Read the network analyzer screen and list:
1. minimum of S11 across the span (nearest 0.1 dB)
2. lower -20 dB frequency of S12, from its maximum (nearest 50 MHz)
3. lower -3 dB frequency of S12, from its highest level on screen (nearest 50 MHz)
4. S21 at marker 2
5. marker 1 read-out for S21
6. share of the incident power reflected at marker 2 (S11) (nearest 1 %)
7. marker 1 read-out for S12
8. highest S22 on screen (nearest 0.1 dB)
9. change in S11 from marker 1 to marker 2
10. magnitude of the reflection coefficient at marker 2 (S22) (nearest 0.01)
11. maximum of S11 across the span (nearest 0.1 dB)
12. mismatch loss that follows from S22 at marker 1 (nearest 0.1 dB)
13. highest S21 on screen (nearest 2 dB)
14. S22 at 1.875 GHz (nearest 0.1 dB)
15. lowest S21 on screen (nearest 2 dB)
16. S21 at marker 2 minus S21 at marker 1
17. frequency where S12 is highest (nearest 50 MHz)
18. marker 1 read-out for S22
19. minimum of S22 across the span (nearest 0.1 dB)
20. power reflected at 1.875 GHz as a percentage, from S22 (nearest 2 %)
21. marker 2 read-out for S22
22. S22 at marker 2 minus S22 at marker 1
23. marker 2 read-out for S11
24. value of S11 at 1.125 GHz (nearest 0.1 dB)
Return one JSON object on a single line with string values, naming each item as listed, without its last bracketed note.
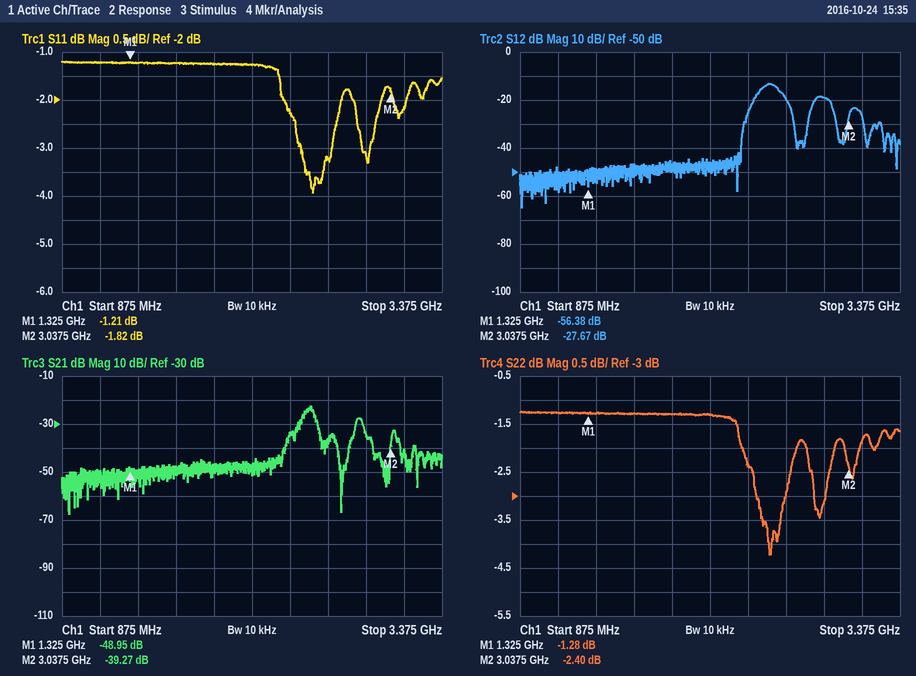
{"minimum of S11 across the span": "-3.9 dB", "lower -20 dB frequency of S12, from its maximum": "2.35 GHz", "lower -3 dB frequency of S12, from its highest level on screen": "2.45 GHz", "S21 at marker 2": "-39.27 dB", "marker 1 read-out for S21": "-48.95 dB", "share of the incident power reflected at marker 2 (S11)": "66 %", "marker 1 read-out for S12": "-56.38 dB", "highest S22 on screen": "-1.2 dB", "change in S11 from marker 1 to marker 2": "-0.61 dB", "magnitude of the reflection coefficient at marker 2 (S22)": "0.76", "maximum of S11 across the span": "-1.2 dB", "mismatch loss that follows from S22 at marker 1": "5.9 dB", "highest S21 on screen": "-22 dB", "S22 at 1.875 GHz": "-1.3 dB", "lowest S21 on screen": "-68 dB", "S21 at marker 2 minus S21 at marker 1": "9.68 dB", "frequency where S12 is highest": "2.50 GHz", "marker 1 read-out for S22": "-1.28 dB", "minimum of S22 across the span": "-4.2 dB", "power reflected at 1.875 GHz as a percentage, from S22": "74 %", "marker 2 read-out for S22": "-2.40 dB", "S22 at marker 2 minus S22 at marker 1": "-1.12 dB", "marker 2 read-out for S11": "-1.82 dB", "value of S11 at 1.125 GHz": "-1.2 dB"}
